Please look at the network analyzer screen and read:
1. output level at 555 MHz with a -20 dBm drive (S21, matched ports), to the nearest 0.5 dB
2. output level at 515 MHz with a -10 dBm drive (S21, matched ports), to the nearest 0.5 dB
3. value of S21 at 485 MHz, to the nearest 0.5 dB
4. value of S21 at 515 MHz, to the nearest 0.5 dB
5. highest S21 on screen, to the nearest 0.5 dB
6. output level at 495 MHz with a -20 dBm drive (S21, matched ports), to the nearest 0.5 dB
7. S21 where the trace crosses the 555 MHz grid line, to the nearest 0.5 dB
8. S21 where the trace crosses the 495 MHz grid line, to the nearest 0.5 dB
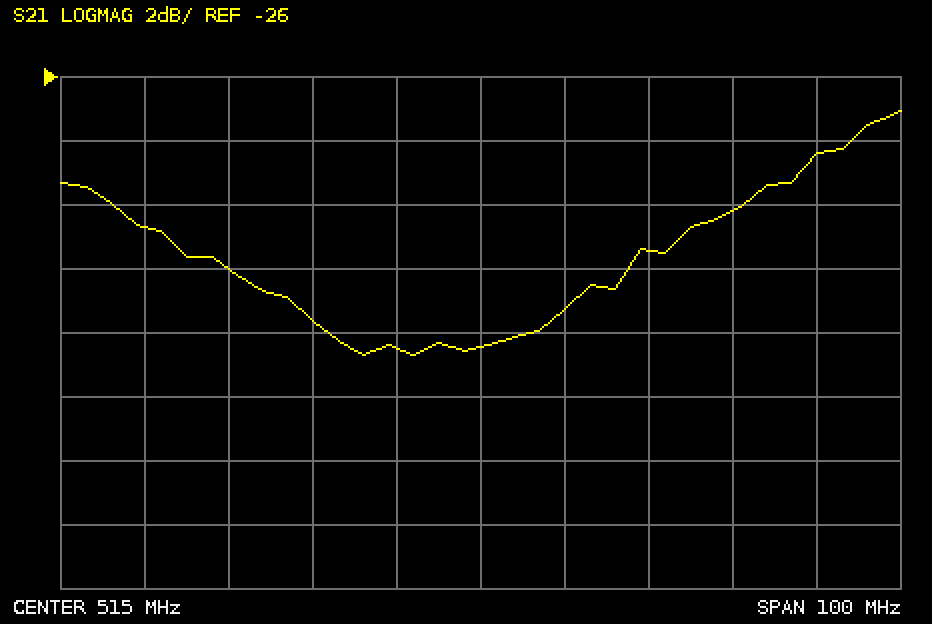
-48.5 dBm
-44.5 dBm
-32.0 dB
-34.5 dB
-27.0 dB
-53.5 dBm
-28.5 dB
-33.5 dB
